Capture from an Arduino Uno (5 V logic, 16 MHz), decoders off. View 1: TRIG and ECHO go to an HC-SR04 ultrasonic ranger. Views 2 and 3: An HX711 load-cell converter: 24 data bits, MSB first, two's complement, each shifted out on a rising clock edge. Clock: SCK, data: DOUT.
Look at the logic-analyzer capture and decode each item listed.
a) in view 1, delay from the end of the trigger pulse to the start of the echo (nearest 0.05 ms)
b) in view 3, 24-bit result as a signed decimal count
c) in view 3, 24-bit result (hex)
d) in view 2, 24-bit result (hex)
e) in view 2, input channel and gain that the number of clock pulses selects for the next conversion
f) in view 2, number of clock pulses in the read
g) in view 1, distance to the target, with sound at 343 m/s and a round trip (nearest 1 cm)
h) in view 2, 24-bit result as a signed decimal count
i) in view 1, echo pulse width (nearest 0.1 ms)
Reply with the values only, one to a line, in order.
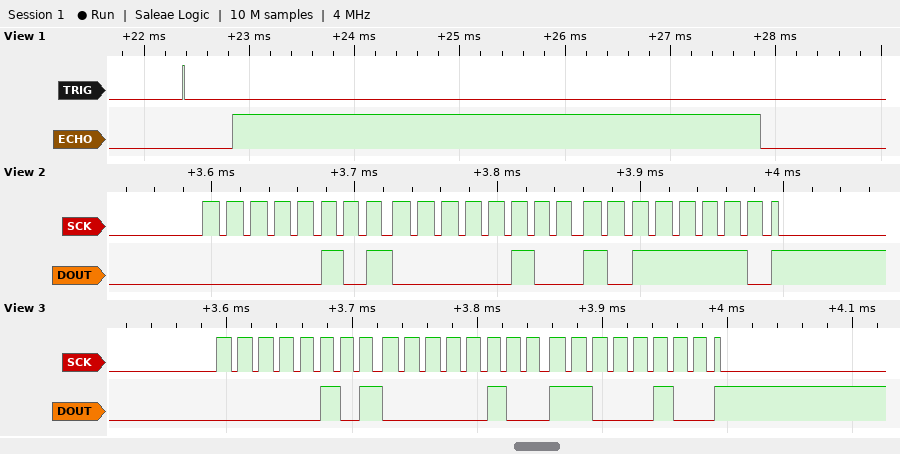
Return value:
0.45 ms
328900
0x0504C4
0x0504BE
channel A, gain 128
25
86 cm
328894
5.0 ms
